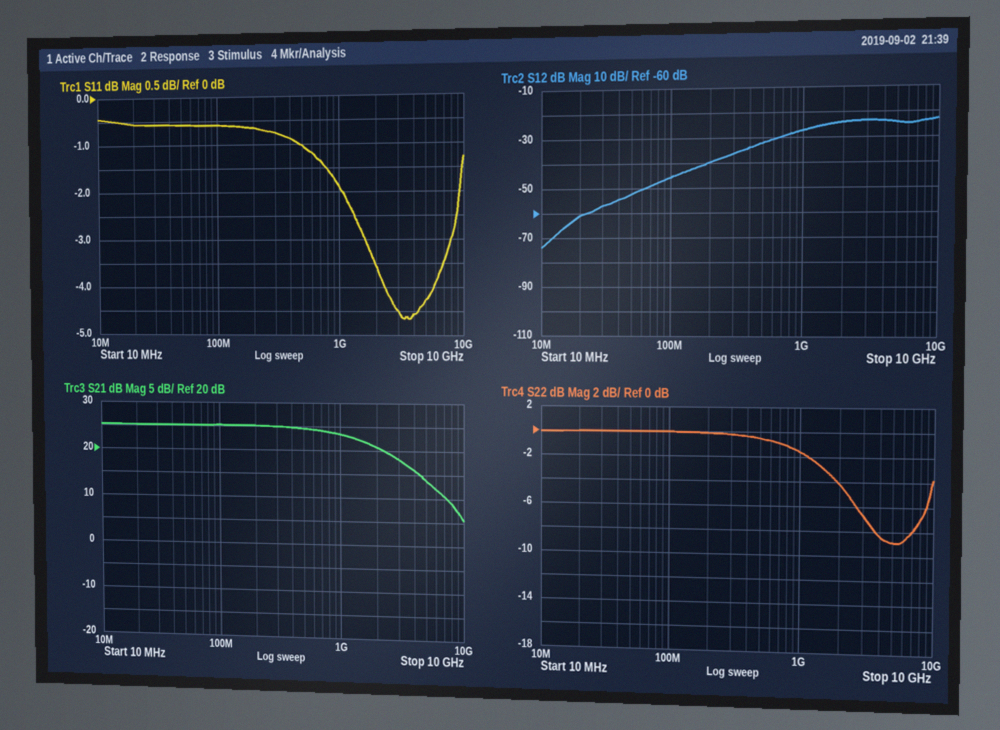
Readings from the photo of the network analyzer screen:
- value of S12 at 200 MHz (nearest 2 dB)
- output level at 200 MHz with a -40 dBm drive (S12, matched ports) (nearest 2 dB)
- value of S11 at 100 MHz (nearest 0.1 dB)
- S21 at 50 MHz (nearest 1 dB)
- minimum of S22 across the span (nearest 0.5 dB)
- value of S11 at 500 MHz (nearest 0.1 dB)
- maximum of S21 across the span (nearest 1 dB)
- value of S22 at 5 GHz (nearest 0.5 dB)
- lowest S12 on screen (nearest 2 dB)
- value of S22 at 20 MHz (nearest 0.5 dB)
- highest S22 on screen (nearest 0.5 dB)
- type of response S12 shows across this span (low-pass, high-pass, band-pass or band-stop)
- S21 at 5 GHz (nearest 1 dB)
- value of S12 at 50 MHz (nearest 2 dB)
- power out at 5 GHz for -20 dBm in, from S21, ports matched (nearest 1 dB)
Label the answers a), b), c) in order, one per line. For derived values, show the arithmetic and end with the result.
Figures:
a) -40 dB
b) -40 dBm + (-40 dB) = -80 dBm
c) -0.6 dB
d) 25 dB
e) -9.0 dB
f) -1.0 dB
g) 25 dB
h) -9.0 dB
i) -74 dB
j) 0.0 dB
k) 0.0 dB
l) high-pass
m) 14 dB
n) -52 dB
o) -20 dBm + (14 dB) = -6 dBm
